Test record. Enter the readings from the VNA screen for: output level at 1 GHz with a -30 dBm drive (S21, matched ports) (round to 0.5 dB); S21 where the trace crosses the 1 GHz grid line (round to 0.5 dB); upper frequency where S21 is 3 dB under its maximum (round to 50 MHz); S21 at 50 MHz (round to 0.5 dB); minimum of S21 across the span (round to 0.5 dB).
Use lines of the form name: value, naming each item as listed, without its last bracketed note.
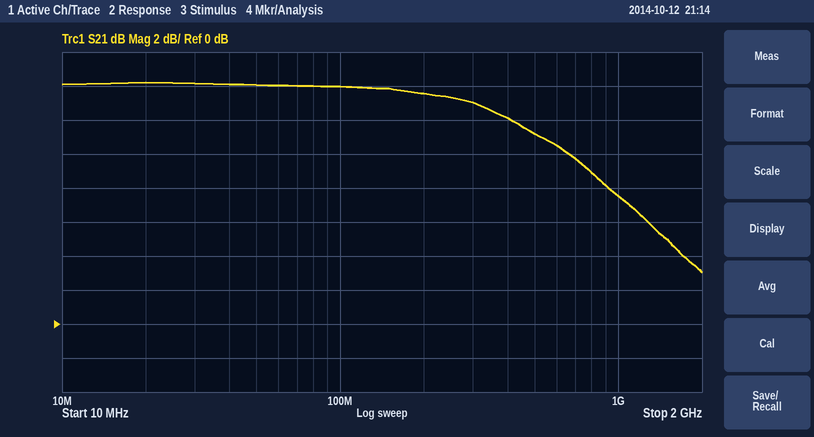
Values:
output level at 1 GHz with a -30 dBm drive (S21, matched ports): -22.5 dBm
S21 where the trace crosses the 1 GHz grid line: 7.5 dB
upper frequency where S21 is 3 dB under its maximum: 500 MHz
S21 at 50 MHz: 14.0 dB
minimum of S21 across the span: 3.0 dB
